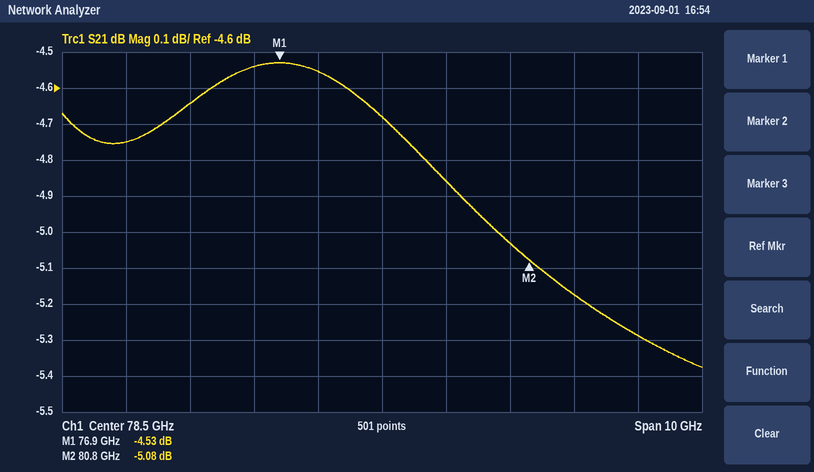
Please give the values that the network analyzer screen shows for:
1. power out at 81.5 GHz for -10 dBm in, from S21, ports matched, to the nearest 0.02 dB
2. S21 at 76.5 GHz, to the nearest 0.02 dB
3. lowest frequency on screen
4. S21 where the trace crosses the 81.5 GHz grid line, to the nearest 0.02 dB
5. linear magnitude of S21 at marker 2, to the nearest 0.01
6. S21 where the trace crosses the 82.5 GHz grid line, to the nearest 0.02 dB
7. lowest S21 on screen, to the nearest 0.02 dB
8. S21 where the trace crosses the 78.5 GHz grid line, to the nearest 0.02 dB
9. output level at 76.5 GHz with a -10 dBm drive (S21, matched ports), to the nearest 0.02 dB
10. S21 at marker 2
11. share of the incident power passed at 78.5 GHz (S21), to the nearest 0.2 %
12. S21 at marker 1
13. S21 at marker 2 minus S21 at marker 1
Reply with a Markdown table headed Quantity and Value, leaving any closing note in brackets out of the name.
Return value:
| Quantity | Value |
|---|---|
| power out at 81.5 GHz for -10 dBm in, from S21, ports matched, to the nearest 0.02 dB | -15.18 dBm |
| S21 at 76.5 GHz, to the nearest 0.02 dB | -4.54 dB |
| lowest frequency on screen | 73.5 GHz |
| S21 where the trace crosses the 81.5 GHz grid line, to the nearest 0.02 dB | -5.18 dB |
| linear magnitude of S21 at marker 2, to the nearest 0.01 | 0.56 |
| S21 where the trace crosses the 82.5 GHz grid line, to the nearest 0.02 dB | -5.28 dB |
| lowest S21 on screen, to the nearest 0.02 dB | -5.38 dB |
| S21 where the trace crosses the 78.5 GHz grid line, to the nearest 0.02 dB | -4.68 dB |
| output level at 76.5 GHz with a -10 dBm drive (S21, matched ports), to the nearest 0.02 dB | -14.54 dBm |
| S21 at marker 2 | -5.08 dB |
| share of the incident power passed at 78.5 GHz (S21), to the nearest 0.2 % | 34.0 % |
| S21 at marker 1 | -4.53 dB |
| S21 at marker 2 minus S21 at marker 1 | -0.55 dB |
